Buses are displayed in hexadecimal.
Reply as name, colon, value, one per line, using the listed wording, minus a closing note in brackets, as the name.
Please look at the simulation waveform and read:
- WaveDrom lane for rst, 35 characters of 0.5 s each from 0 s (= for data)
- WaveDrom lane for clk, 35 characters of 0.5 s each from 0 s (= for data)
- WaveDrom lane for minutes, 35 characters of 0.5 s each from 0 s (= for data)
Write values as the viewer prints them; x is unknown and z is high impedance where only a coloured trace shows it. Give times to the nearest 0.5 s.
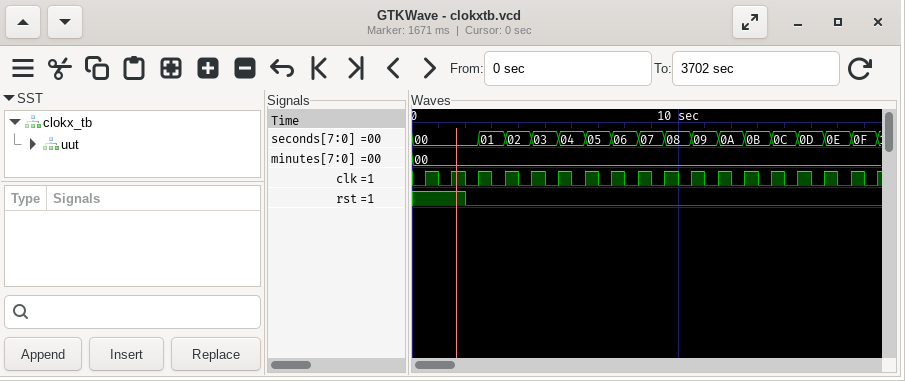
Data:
WaveDrom lane for rst, 35 characters of 0.5 s each from 0 s: {name: 'rst', wave: '1...0..............................'}
WaveDrom lane for clk, 35 characters of 0.5 s each from 0 s: {name: 'clk', wave: '01010101010101010101010101010101010'}
WaveDrom lane for minutes, 35 characters of 0.5 s each from 0 s: {name: 'minutes', wave: '=..................................', data: '00'}
